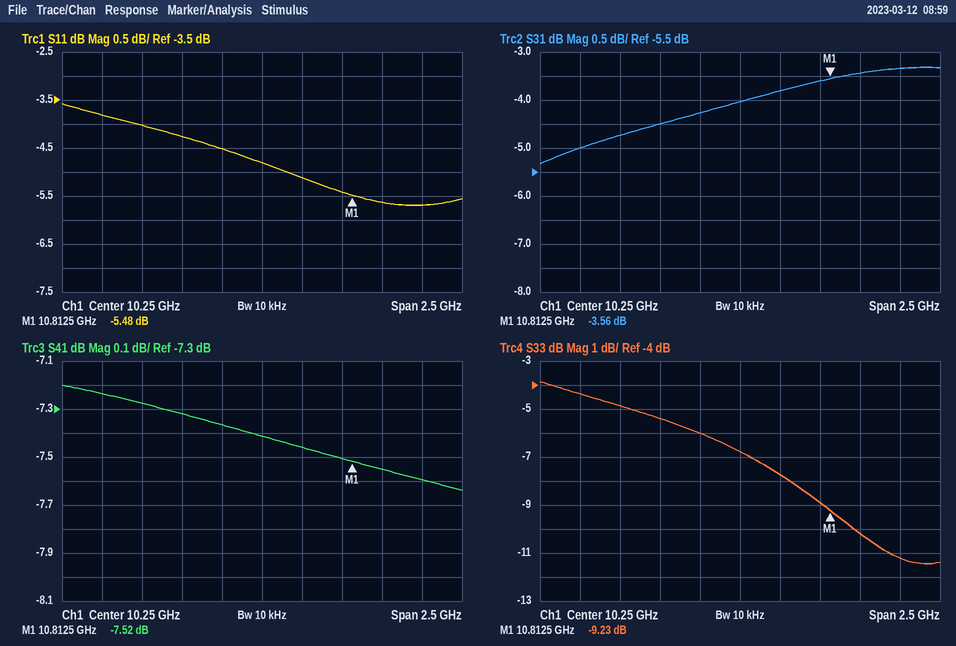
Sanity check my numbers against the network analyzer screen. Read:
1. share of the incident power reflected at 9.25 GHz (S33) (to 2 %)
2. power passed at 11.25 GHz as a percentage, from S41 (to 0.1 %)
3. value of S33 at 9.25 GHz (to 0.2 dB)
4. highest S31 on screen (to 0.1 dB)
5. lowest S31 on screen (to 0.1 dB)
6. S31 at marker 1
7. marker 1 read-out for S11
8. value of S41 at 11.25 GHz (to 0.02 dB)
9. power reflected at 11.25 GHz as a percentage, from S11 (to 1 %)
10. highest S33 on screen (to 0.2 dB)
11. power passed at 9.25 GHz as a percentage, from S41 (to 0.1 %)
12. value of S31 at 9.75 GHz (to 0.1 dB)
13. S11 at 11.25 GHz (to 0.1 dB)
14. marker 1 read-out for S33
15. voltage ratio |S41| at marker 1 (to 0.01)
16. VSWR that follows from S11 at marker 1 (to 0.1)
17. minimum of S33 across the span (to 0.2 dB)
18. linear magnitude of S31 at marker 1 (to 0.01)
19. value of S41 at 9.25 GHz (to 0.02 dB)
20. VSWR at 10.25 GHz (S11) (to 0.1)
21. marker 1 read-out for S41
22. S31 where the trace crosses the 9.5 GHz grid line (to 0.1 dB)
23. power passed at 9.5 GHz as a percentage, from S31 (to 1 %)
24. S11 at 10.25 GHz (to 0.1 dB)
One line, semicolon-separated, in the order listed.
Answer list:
36 %; 17.4 %; -4.4 dB; -3.3 dB; -5.3 dB; -3.56 dB; -5.48 dB; -7.60 dB; 27 %; -3.8 dB; 18.9 %; -4.5 dB; -5.7 dB; -9.23 dB; 0.42; 3.3; -11.4 dB; 0.66; -7.24 dB; 3.7; -7.52 dB; -4.7 dB; 34 %; -4.8 dB
